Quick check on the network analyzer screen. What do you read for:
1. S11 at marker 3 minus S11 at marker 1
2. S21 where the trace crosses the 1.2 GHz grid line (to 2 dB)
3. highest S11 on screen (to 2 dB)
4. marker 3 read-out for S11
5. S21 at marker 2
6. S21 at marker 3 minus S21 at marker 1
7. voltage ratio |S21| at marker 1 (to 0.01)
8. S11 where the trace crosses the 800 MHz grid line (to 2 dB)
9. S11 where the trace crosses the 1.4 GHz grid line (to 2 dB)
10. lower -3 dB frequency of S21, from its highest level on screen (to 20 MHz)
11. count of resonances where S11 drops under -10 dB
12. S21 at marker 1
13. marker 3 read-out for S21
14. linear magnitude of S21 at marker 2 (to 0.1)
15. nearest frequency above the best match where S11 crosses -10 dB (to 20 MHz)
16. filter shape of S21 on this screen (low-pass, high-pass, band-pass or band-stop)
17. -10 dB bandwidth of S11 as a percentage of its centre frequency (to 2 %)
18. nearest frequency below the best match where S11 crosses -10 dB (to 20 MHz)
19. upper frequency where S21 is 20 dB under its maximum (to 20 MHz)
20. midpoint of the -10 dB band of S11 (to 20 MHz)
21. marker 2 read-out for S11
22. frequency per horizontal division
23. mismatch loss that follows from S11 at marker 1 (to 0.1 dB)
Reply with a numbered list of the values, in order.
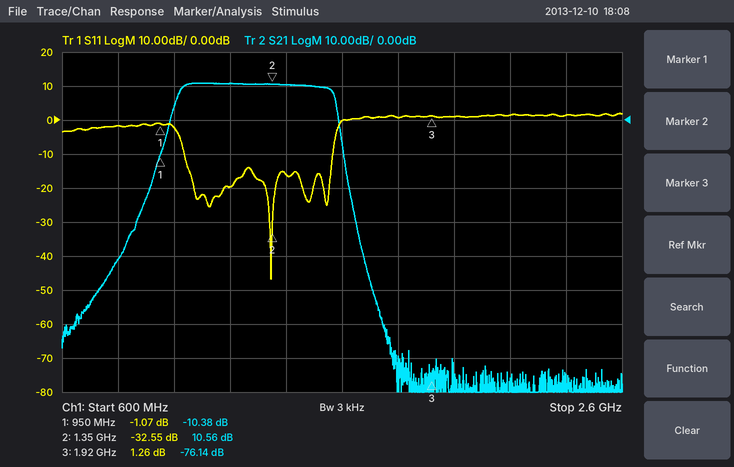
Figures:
1. 2.33 dB
2. 10 dB
3. 2 dB
4. 1.26 dB
5. 10.56 dB
6. -65.76 dB
7. 0.30
8. -2 dB
9. -16 dB
10. 1.02 GHz
11. 4
12. -10.38 dB
13. -76.14 dB
14. 3.4
15. 1.56 GHz
16. band-pass
17. 40 %
18. 1.04 GHz
19. 1.60 GHz
20. 1.30 GHz
21. -32.55 dB
22. 200 MHz
23. 6.6 dB
